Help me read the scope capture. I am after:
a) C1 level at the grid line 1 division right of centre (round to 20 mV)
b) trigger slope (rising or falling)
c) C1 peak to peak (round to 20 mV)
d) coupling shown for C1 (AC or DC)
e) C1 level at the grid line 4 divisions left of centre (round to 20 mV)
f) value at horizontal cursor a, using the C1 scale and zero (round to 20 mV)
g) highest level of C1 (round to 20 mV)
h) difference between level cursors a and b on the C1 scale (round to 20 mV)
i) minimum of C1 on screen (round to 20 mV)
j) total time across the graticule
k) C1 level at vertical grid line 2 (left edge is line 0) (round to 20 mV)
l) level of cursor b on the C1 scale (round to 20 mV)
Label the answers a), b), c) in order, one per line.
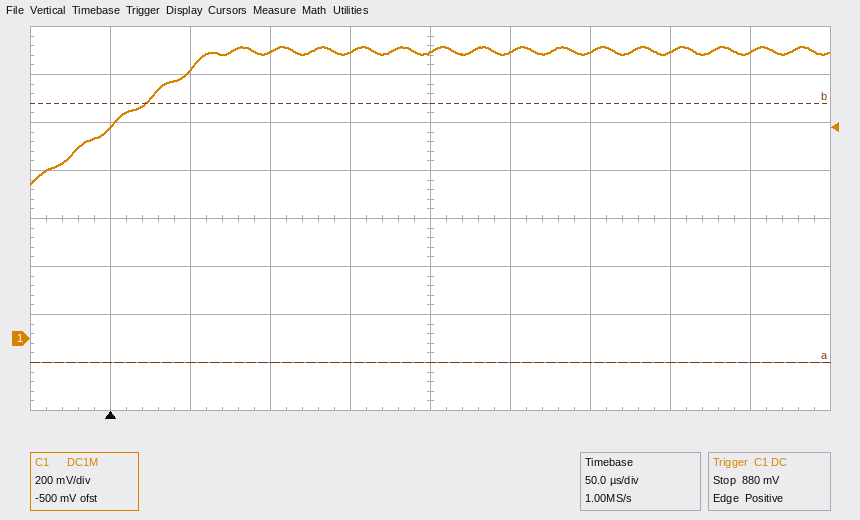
a) 1.20 V
b) rising
c) 580 mV
d) DC
e) 880 mV
f) -100 mV
g) 1.22 V
h) 1.08 V
i) 640 mV
j) 500 µs
k) 1.12 V
l) 980 mV
